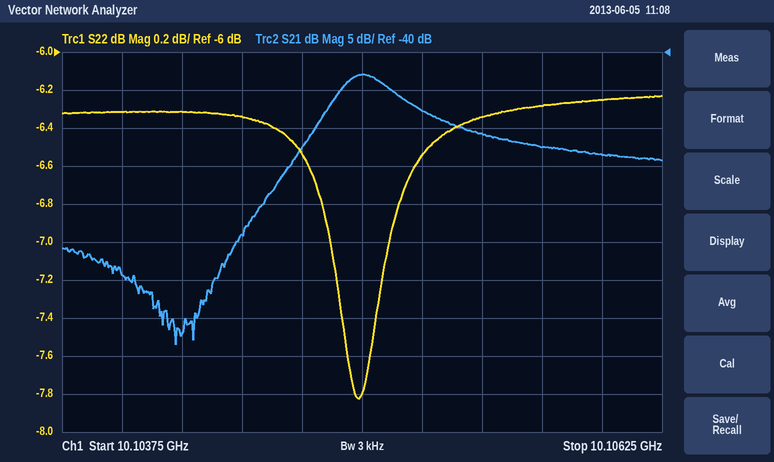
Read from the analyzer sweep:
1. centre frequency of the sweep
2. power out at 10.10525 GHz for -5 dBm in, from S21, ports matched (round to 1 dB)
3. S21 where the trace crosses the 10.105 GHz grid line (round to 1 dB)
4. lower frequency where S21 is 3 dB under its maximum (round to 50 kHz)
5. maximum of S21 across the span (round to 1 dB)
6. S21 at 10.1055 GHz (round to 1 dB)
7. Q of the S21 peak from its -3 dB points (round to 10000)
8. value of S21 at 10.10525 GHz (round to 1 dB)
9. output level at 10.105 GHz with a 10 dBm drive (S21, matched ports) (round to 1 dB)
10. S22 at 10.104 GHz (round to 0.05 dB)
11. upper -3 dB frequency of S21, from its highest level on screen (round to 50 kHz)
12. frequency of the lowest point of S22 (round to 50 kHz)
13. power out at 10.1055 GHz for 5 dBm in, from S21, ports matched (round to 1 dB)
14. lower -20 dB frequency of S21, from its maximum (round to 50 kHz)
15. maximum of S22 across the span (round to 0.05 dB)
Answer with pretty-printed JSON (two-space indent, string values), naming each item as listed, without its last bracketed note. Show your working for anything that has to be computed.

{
  "centre frequency of the sweep": "10.105 GHz",
  "power out at 10.10525 GHz for -5 dBm in, from S21, ports matched": "-5 dBm + (-48 dB) = -53 dBm",
  "S21 where the trace crosses the 10.105 GHz grid line": "-43 dB",
  "lower frequency where S21 is 3 dB under its maximum": "10.10490 GHz",
  "maximum of S21 across the span": "-43 dB",
  "S21 at 10.1055 GHz": "-51 dB",
  "Q of the S21 peak from its -3 dB points": "10.105 GHz / 250 kHz ≈ 40420, so 40000 to the nearest 10000",
  "value of S21 at 10.10525 GHz": "-48 dB",
  "output level at 10.105 GHz with a 10 dBm drive (S21, matched ports)": "10 dBm + (-43 dB) = -33 dBm",
  "S22 at 10.104 GHz": "-6.30 dB",
  "upper -3 dB frequency of S21, from its highest level on screen": "10.10515 GHz",
  "frequency of the lowest point of S22": "10.10500 GHz",
  "power out at 10.1055 GHz for 5 dBm in, from S21, ports matched": "5 dBm + (-51 dB) = -46 dBm",
  "lower -20 dB frequency of S21, from its maximum": "10.10450 GHz",
  "maximum of S22 across the span": "-6.25 dB"
}
